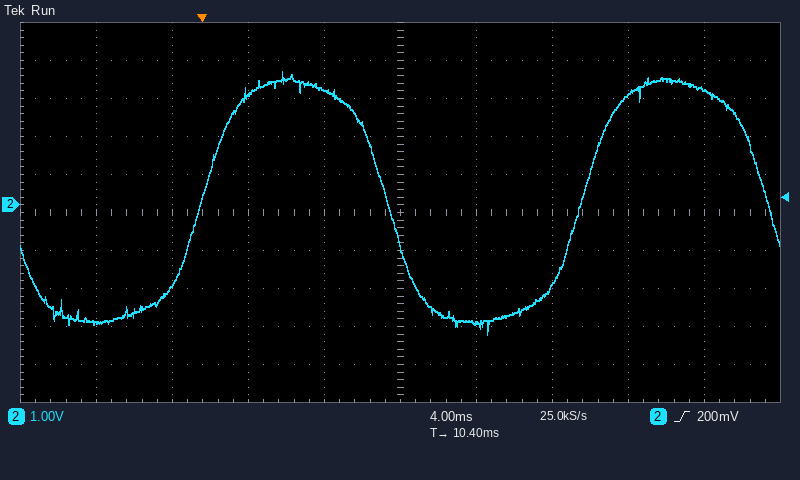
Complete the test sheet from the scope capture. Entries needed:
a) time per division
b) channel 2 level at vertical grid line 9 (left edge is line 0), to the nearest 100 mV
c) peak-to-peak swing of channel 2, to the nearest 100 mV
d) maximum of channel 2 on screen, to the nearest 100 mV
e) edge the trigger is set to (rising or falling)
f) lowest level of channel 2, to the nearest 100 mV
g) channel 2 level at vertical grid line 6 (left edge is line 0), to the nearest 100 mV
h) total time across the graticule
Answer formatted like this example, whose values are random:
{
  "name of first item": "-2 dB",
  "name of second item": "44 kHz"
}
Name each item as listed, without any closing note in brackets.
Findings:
{
  "time per division": "4 ms",
  "channel 2 level at vertical grid line 9 (left edge is line 0), to the nearest 100 mV": "3.0 V",
  "peak-to-peak swing of channel 2, to the nearest 100 mV": "6.9 V",
  "maximum of channel 2 on screen, to the nearest 100 mV": "3.5 V",
  "edge the trigger is set to": "rising",
  "lowest level of channel 2, to the nearest 100 mV": "-3.4 V",
  "channel 2 level at vertical grid line 6 (left edge is line 0), to the nearest 100 mV": "-3.1 V",
  "total time across the graticule": "40 ms"
}
